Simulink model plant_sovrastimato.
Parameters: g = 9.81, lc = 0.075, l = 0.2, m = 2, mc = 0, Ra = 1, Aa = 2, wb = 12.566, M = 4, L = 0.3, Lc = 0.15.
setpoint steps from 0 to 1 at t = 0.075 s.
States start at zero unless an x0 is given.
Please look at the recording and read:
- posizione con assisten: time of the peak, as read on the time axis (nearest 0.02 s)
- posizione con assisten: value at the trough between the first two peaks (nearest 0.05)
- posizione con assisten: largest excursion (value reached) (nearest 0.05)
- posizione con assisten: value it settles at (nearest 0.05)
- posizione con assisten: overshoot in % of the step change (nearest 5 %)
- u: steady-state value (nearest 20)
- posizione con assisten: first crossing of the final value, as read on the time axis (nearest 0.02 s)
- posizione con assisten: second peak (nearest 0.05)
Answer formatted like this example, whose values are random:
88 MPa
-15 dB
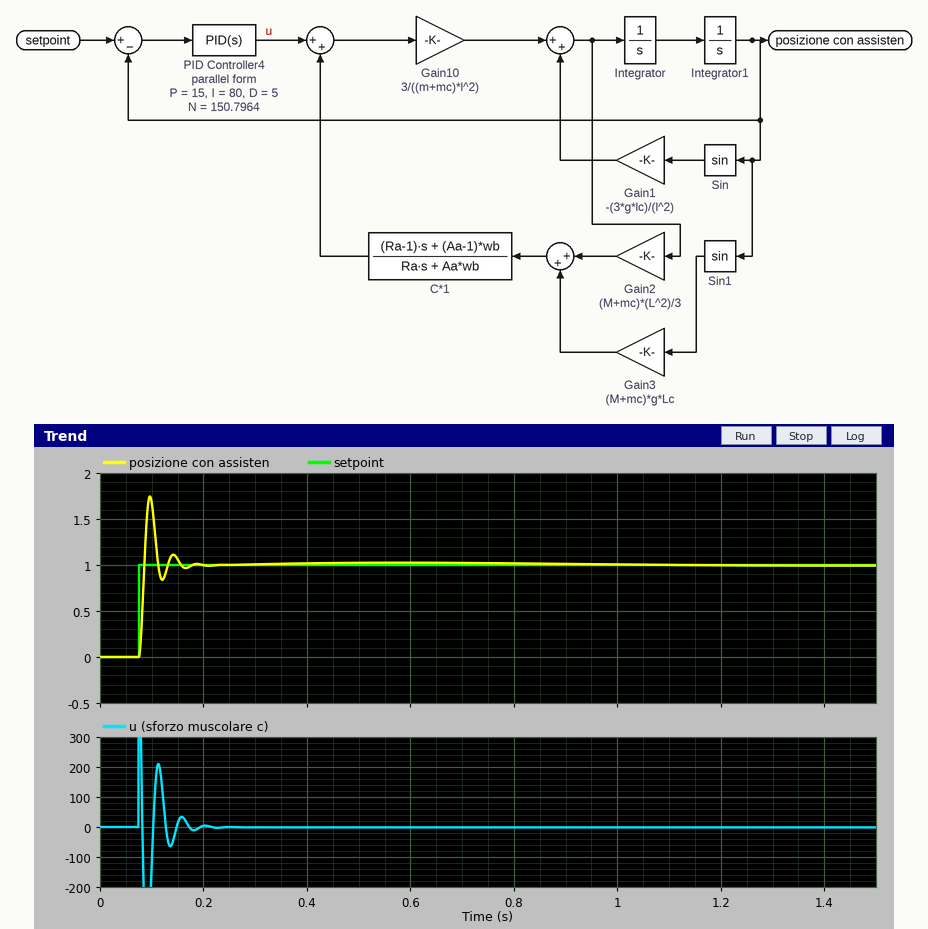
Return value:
0.10 s
0.85
1.75
1.00
75 %
0
0.08 s
1.10
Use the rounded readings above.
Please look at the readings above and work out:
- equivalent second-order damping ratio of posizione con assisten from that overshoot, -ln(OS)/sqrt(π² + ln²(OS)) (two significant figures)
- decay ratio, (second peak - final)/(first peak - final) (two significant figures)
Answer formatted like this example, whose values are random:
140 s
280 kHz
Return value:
0.091
0.13
